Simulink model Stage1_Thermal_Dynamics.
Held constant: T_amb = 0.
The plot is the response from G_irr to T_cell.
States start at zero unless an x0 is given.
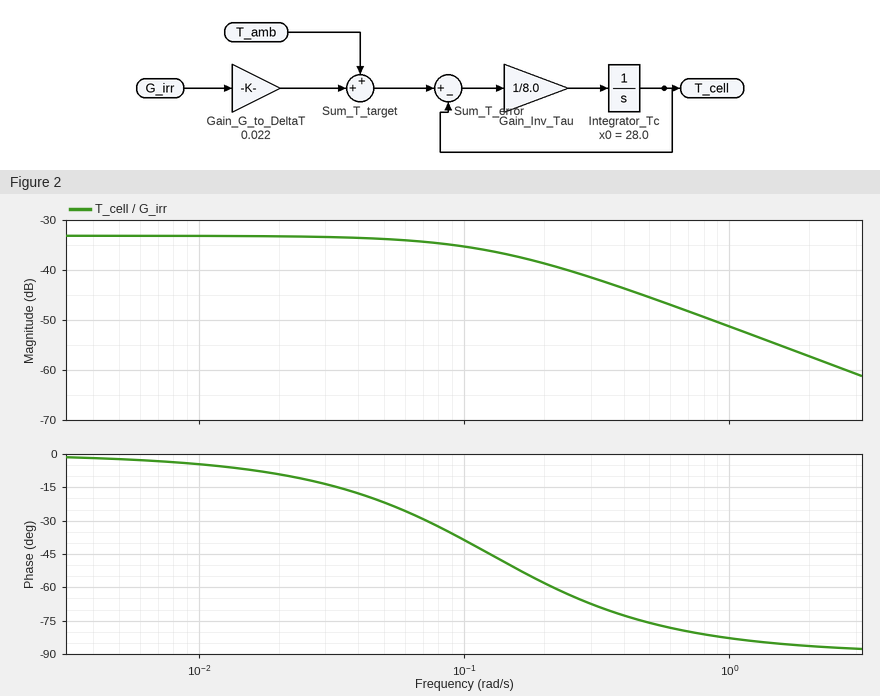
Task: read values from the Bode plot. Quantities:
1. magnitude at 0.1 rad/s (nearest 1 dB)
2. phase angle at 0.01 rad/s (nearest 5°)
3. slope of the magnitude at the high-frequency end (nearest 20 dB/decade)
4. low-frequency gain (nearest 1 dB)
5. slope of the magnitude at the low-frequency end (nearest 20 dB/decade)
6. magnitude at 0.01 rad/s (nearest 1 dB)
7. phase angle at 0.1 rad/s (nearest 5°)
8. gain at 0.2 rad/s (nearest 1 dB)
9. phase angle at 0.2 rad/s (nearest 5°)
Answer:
-35 dB
-5°
-20 dB/decade
-33 dB
0 dB/decade
-33 dB
-40°
-39 dB
-60°
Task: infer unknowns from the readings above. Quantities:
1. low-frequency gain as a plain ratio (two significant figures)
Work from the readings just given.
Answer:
0.022
